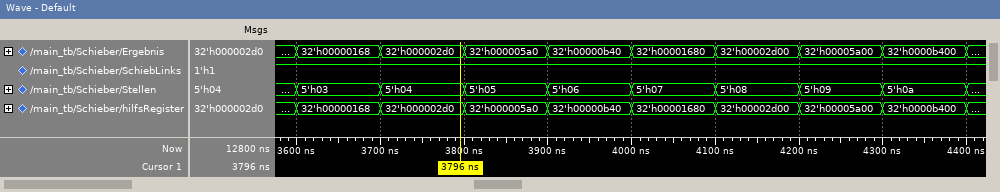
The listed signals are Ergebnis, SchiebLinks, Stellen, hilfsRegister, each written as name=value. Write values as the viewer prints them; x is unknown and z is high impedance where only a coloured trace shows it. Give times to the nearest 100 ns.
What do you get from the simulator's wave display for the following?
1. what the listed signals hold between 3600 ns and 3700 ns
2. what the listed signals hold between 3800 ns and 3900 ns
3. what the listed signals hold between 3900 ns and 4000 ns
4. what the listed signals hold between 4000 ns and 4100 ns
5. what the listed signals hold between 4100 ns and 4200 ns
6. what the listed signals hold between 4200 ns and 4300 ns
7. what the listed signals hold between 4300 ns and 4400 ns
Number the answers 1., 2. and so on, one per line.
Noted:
1. Ergebnis=32'h00000168, SchiebLinks=1, Stellen=5'h03, hilfsRegister=32'h00000168
2. Ergebnis=32'h000005a0, SchiebLinks=1, Stellen=5'h05, hilfsRegister=32'h000005a0
3. Ergebnis=32'h00000b40, SchiebLinks=1, Stellen=5'h06, hilfsRegister=32'h00000b40
4. Ergebnis=32'h00001680, SchiebLinks=1, Stellen=5'h07, hilfsRegister=32'h00001680
5. Ergebnis=32'h00002d00, SchiebLinks=1, Stellen=5'h08, hilfsRegister=32'h00002d00
6. Ergebnis=32'h00005a00, SchiebLinks=1, Stellen=5'h09, hilfsRegister=32'h00005a00
7. Ergebnis=32'h0000b400, SchiebLinks=1, Stellen=5'h0a, hilfsRegister=32'h0000b400
